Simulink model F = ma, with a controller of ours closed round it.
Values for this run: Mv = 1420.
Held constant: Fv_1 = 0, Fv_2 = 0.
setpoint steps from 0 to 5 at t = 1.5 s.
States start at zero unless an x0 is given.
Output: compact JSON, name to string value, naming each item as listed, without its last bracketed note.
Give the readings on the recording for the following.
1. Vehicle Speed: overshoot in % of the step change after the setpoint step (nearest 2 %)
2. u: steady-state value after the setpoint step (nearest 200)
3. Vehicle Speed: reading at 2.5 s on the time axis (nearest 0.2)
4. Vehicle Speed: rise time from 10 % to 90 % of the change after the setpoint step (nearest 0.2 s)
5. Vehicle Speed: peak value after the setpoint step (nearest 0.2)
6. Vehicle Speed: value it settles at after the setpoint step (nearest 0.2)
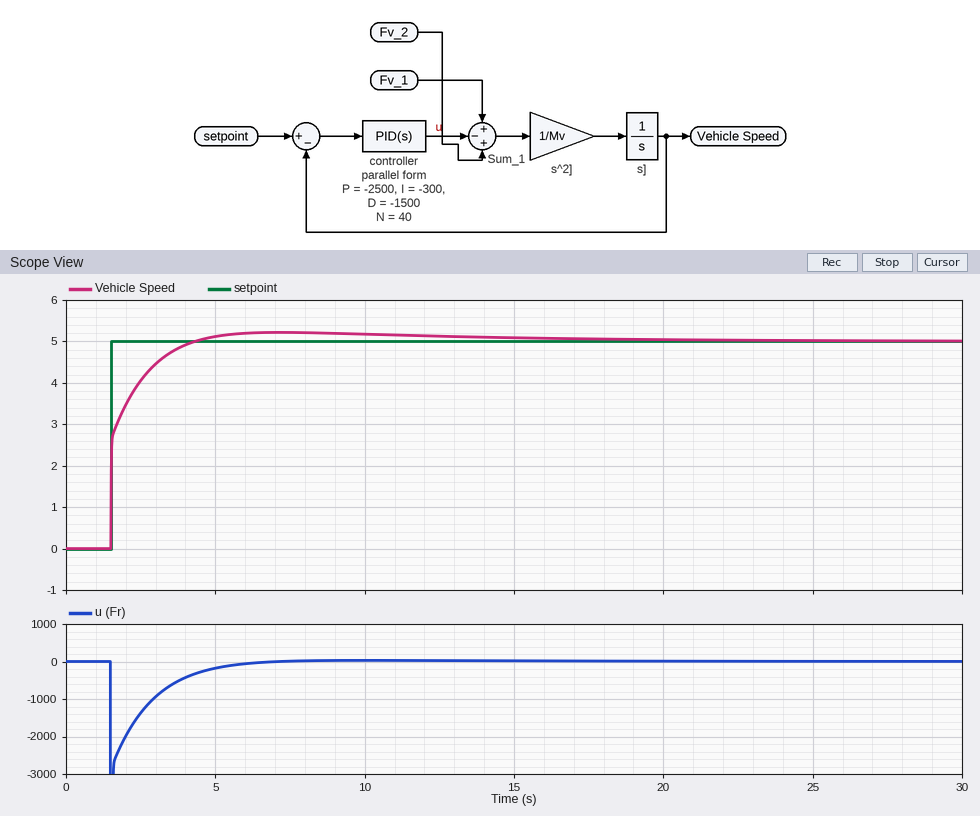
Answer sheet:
{"Vehicle Speed: overshoot in % of the step change after the setpoint step": "4 %", "u: steady-state value after the setpoint step": "0", "Vehicle Speed: reading at 2.5 s on the time axis": "4.0", "Vehicle Speed: rise time from 10 % to 90 % of the change after the setpoint step": "1.6 s", "Vehicle Speed: peak value after the setpoint step": "5.2", "Vehicle Speed: value it settles at after the setpoint step": "5.0"}
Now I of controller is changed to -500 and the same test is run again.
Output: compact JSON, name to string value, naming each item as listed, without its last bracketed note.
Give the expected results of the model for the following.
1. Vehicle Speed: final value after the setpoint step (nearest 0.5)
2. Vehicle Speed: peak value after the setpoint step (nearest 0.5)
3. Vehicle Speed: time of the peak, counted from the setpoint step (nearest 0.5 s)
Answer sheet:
{"Vehicle Speed: final value after the setpoint step": "5.0", "Vehicle Speed: peak value after the setpoint step": "5.5", "Vehicle Speed: time of the peak, counted from the setpoint step": "5.0 s"}
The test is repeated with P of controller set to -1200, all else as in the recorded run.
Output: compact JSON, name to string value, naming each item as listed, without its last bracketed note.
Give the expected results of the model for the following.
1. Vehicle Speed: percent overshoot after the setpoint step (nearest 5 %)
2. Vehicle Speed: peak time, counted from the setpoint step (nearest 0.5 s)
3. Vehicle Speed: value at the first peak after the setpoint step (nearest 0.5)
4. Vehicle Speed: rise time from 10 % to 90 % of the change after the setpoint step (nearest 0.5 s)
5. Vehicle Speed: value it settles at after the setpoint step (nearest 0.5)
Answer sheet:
{"Vehicle Speed: percent overshoot after the setpoint step": "10 %", "Vehicle Speed: peak time, counted from the setpoint step": "7.0 s", "Vehicle Speed: value at the first peak after the setpoint step": "5.5", "Vehicle Speed: rise time from 10 % to 90 % of the change after the setpoint step": "2.5 s", "Vehicle Speed: value it settles at after the setpoint step": "5.0"}
